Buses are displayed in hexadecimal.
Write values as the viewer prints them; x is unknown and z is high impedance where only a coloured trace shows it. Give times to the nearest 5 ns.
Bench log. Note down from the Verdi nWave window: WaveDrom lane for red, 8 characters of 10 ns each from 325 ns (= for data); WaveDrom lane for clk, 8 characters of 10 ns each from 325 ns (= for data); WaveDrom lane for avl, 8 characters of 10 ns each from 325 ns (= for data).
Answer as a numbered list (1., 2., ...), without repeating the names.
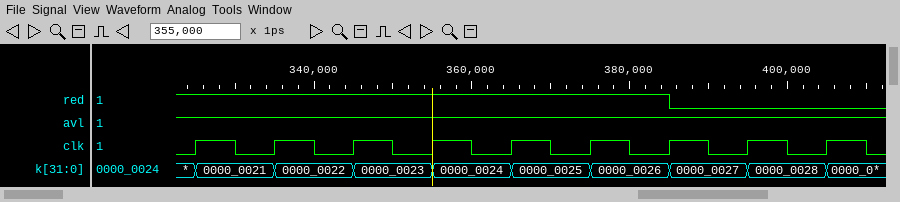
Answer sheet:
1. {name: 'red', wave: '1.....0.'}
2. {name: 'clk', wave: 'p.......'}
3. {name: 'avl', wave: '1.......'}
